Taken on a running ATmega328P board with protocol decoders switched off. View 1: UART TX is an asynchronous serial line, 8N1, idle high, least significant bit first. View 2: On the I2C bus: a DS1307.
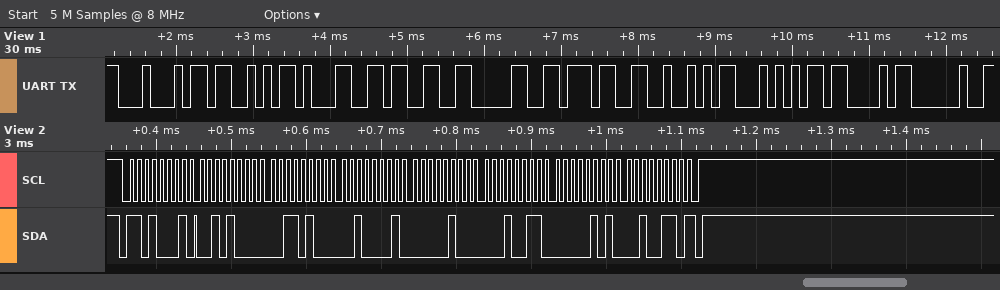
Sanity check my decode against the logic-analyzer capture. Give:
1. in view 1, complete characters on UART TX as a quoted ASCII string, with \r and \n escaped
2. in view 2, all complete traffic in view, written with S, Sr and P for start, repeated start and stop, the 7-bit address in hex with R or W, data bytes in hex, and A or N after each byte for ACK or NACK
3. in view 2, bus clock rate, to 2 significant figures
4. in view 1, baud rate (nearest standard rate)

"DS1307RTC "
S 68R A 28 A 34 A 21 A 04 A 13 A 05 A 26 N P
100 kHz
9600 baud
